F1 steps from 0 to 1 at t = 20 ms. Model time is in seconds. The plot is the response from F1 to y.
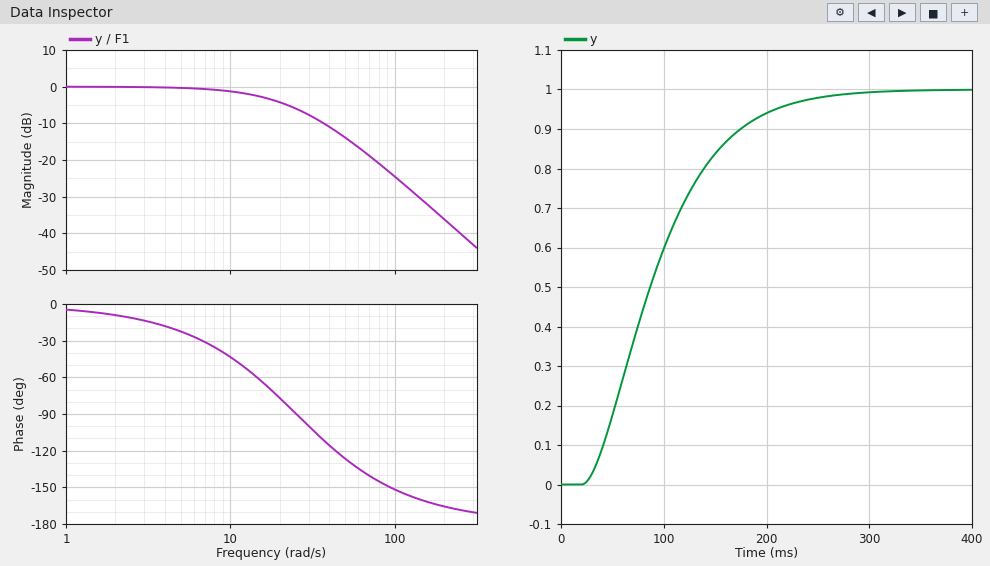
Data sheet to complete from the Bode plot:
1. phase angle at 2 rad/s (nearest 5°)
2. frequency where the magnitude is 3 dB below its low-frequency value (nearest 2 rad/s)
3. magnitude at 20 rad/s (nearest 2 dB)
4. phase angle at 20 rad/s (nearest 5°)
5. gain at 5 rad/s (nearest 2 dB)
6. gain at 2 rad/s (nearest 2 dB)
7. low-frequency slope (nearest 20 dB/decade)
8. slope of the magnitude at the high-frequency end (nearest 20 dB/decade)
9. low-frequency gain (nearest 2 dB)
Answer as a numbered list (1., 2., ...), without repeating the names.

1. -10°
2. 16 rad/s
3. -4 dB
4. -75°
5. 0 dB
6. 0 dB
7. 0 dB/decade
8. -40 dB/decade
9. 0 dB
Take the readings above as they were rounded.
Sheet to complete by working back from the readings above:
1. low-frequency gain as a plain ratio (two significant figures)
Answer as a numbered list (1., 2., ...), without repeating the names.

1. 1.0
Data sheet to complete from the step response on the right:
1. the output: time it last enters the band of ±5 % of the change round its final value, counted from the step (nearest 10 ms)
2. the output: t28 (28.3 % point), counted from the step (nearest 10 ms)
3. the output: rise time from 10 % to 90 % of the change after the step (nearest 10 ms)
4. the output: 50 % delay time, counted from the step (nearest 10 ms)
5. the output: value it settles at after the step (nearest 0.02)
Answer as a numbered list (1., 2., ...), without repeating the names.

1. 190 ms
2. 40 ms
3. 130 ms
4. 70 ms
5. 1.00
